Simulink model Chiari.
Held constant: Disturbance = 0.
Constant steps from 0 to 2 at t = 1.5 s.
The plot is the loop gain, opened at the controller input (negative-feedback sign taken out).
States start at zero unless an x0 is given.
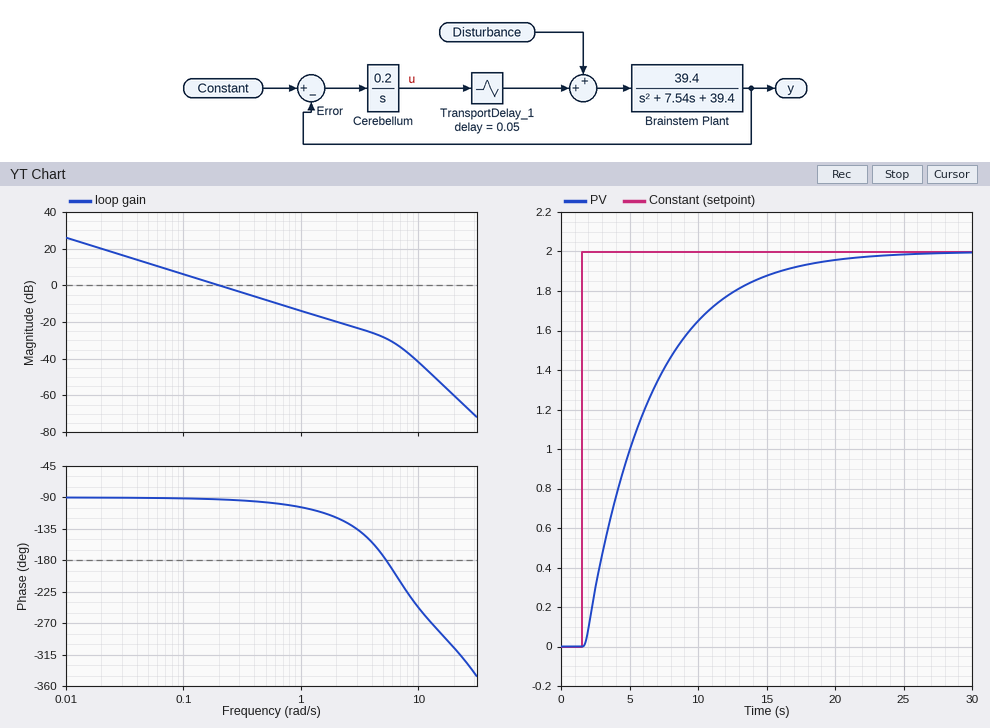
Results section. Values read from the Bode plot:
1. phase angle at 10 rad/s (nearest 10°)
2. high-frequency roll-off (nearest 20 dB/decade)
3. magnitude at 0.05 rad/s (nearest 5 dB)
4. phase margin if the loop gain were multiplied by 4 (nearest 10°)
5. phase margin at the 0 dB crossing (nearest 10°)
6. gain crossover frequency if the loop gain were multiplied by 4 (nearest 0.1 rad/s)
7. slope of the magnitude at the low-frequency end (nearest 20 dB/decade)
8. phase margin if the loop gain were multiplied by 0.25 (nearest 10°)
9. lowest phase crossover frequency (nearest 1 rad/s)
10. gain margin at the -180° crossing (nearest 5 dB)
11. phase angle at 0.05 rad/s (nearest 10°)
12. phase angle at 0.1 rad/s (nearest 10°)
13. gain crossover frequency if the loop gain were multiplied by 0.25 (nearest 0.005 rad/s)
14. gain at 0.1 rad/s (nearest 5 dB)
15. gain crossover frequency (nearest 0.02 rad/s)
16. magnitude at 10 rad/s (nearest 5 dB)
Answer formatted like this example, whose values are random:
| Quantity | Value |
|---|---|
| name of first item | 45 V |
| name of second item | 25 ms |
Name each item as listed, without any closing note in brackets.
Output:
| Quantity | Value |
|---|---|
| phase angle at 10 rad/s | -250° |
| high-frequency roll-off | -60 dB/decade |
| magnitude at 0.05 rad/s | 10 dB |
| phase margin if the loop gain were multiplied by 4 | 80° |
| phase margin at the 0 dB crossing | 90° |
| gain crossover frequency if the loop gain were multiplied by 4 | 0.8 rad/s |
| slope of the magnitude at the low-frequency end | -20 dB/decade |
| phase margin if the loop gain were multiplied by 0.25 | 90° |
| lowest phase crossover frequency | 5 rad/s |
| gain margin at the -180° crossing | 30 dB |
| phase angle at 0.05 rad/s | -90° |
| phase angle at 0.1 rad/s | -90° |
| gain crossover frequency if the loop gain were multiplied by 0.25 | 0.050 rad/s |
| gain at 0.1 rad/s | 5 dB |
| gain crossover frequency | 0.20 rad/s |
| magnitude at 10 rad/s | -40 dB |
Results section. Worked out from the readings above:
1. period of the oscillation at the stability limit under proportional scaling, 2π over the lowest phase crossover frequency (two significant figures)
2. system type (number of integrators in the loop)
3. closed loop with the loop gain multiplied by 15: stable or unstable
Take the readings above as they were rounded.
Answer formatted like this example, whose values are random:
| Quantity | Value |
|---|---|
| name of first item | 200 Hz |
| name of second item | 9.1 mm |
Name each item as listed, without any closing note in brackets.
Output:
| Quantity | Value |
|---|---|
| period of the oscillation at the stability limit under proportional scaling, 2π over the lowest phase crossover frequency | 1.3 s |
| system type | 1 |
| closed loop with the loop gain multiplied by 15: stable or unstable | stable |
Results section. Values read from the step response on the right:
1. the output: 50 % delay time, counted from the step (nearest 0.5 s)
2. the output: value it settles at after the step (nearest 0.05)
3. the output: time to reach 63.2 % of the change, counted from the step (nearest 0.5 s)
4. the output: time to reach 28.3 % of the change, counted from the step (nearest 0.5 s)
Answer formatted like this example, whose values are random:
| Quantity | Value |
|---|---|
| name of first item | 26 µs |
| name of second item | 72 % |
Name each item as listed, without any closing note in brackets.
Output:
| Quantity | Value |
|---|---|
| the output: 50 % delay time, counted from the step | 3.5 s |
| the output: value it settles at after the step | 2.00 |
| the output: time to reach 63.2 % of the change, counted from the step | 5.0 s |
| the output: time to reach 28.3 % of the change, counted from the step | 2.0 s |
